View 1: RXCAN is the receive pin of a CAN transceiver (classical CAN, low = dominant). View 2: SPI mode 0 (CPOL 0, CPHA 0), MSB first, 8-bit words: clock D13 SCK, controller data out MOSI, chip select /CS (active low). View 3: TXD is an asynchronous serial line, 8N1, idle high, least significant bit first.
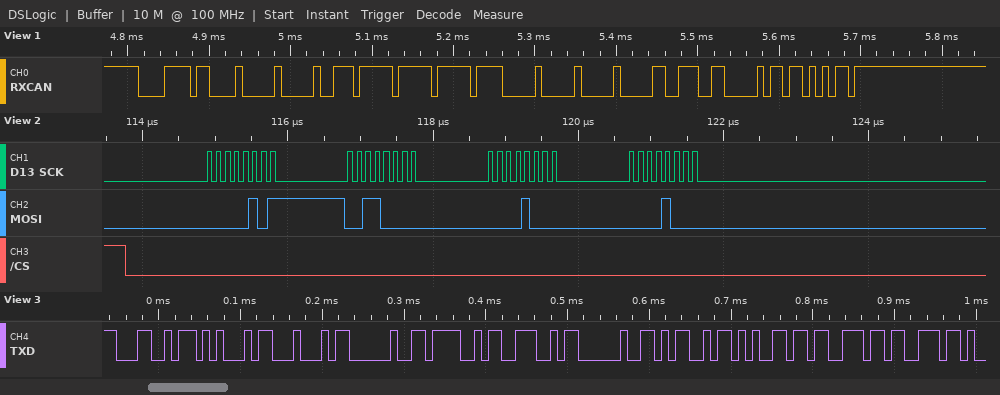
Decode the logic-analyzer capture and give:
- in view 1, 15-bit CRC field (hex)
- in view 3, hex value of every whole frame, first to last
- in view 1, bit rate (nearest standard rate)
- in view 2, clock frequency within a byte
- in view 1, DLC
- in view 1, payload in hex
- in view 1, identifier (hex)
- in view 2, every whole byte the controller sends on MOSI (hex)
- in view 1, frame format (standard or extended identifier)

0x06D5
4C 45 44 20 4F 4E 20 4D 65 73 73
125 kbit/s
8 MHz
8
00 77 FF FF 00 00 09 CC
0x0F6
05 30 08 08
standard
